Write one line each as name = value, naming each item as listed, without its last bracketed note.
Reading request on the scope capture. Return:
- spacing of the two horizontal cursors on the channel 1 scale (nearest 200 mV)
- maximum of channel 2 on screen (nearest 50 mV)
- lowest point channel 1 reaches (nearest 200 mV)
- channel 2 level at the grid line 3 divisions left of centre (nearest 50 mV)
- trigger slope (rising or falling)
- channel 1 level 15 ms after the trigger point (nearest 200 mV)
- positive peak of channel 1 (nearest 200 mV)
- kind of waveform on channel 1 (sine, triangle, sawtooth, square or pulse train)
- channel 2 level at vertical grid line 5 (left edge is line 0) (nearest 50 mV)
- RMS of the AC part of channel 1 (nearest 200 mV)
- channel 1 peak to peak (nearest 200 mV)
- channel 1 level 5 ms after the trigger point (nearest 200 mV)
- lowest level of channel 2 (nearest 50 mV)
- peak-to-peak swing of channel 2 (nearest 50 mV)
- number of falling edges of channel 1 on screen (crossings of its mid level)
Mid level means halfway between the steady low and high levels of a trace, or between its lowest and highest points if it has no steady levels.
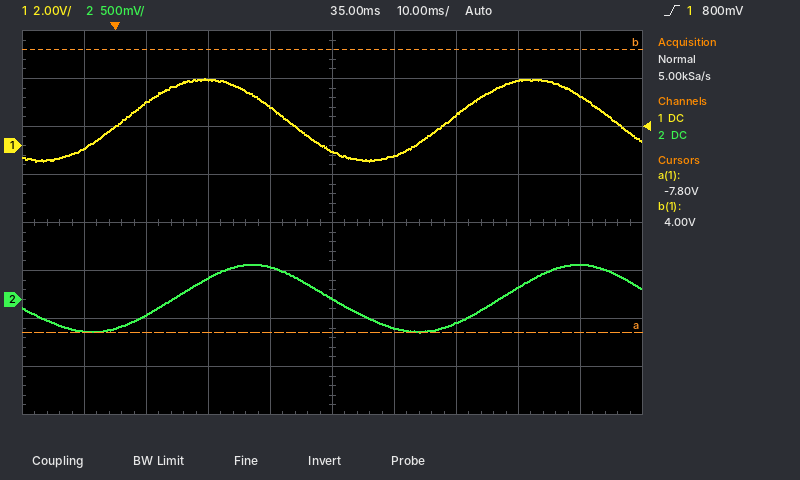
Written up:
spacing of the two horizontal cursors on the channel 1 scale = 11.8 V
maximum of channel 2 on screen = 350 mV
lowest point channel 1 reaches = -600 mV
channel 2 level at the grid line 3 divisions left of centre = -150 mV
trigger slope = rising
channel 1 level 15 ms after the trigger point = 2.8 V
positive peak of channel 1 = 2.8 V
kind of waveform on channel 1 = sine
channel 2 level at vertical grid line 5 (left edge is line 0) = 0 mV
RMS of the AC part of channel 1 = 1.2 V
channel 1 peak to peak = 3.4 V
channel 1 level 5 ms after the trigger point = 1.8 V
lowest level of channel 2 = -350 mV
peak-to-peak swing of channel 2 = 700 mV
number of falling edges of channel 1 on screen = 2
